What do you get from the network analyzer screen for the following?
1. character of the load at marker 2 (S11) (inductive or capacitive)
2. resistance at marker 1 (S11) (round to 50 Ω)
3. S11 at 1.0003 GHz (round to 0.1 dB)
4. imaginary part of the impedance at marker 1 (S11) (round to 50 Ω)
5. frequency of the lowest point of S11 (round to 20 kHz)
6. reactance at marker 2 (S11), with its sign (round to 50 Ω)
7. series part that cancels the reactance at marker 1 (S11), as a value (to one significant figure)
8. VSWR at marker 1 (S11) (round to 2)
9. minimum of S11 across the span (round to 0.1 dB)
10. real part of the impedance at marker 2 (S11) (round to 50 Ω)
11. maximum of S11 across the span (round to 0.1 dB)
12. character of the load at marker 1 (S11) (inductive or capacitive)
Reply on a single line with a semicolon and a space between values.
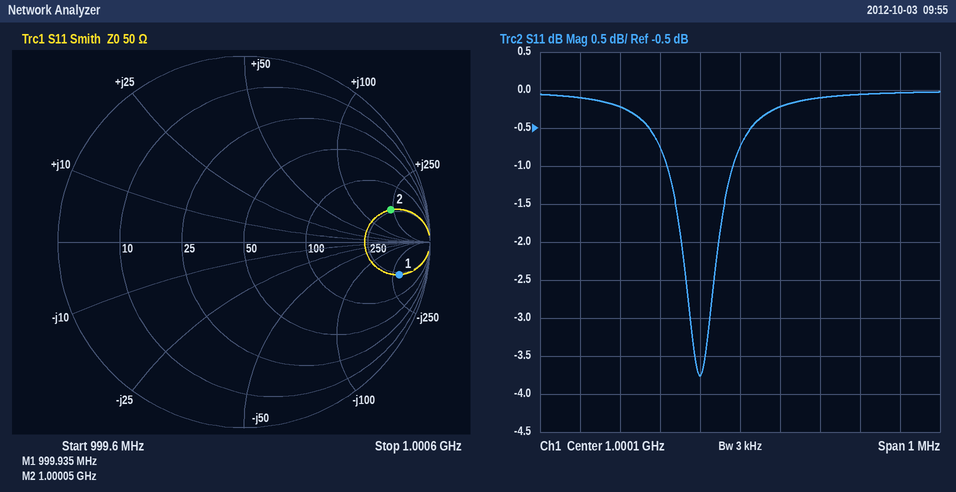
inductive; 250 Ω; -0.1 dB; -300 Ω; 1.00000 GHz; +250 Ω; 50 nH; 12; -3.8 dB; 250 Ω; 0.0 dB; capacitive
